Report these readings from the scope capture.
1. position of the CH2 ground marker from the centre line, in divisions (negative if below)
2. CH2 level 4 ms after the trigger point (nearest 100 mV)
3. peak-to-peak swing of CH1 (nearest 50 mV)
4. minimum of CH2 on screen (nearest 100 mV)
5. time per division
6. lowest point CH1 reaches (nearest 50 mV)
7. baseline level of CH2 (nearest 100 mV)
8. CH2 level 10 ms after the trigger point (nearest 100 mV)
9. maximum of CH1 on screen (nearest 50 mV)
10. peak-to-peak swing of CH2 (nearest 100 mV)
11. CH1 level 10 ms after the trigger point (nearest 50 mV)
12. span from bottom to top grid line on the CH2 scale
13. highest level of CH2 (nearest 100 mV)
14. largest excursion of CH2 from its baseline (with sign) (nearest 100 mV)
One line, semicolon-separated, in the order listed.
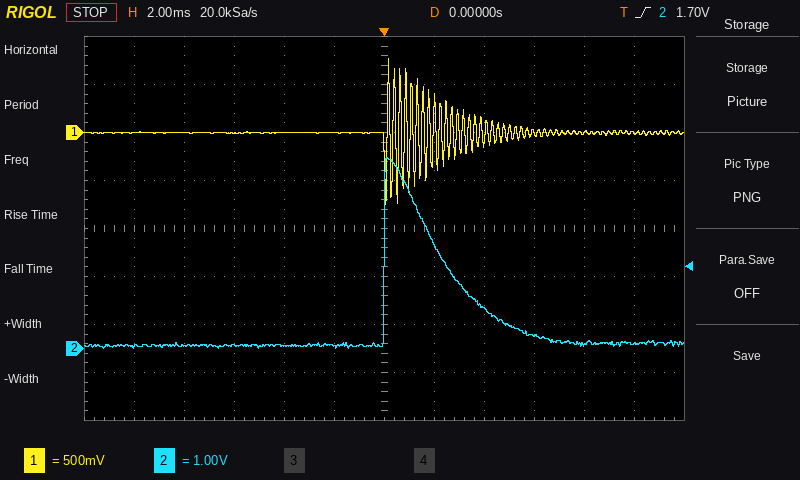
-2.5 div; 800 mV; 1.50 V; 0.0 V; 2 ms; -750 mV; 100 mV; 100 mV; 750 mV; 4.0 V; 0 mV; 8 V; 4.0 V; +3.9 V
